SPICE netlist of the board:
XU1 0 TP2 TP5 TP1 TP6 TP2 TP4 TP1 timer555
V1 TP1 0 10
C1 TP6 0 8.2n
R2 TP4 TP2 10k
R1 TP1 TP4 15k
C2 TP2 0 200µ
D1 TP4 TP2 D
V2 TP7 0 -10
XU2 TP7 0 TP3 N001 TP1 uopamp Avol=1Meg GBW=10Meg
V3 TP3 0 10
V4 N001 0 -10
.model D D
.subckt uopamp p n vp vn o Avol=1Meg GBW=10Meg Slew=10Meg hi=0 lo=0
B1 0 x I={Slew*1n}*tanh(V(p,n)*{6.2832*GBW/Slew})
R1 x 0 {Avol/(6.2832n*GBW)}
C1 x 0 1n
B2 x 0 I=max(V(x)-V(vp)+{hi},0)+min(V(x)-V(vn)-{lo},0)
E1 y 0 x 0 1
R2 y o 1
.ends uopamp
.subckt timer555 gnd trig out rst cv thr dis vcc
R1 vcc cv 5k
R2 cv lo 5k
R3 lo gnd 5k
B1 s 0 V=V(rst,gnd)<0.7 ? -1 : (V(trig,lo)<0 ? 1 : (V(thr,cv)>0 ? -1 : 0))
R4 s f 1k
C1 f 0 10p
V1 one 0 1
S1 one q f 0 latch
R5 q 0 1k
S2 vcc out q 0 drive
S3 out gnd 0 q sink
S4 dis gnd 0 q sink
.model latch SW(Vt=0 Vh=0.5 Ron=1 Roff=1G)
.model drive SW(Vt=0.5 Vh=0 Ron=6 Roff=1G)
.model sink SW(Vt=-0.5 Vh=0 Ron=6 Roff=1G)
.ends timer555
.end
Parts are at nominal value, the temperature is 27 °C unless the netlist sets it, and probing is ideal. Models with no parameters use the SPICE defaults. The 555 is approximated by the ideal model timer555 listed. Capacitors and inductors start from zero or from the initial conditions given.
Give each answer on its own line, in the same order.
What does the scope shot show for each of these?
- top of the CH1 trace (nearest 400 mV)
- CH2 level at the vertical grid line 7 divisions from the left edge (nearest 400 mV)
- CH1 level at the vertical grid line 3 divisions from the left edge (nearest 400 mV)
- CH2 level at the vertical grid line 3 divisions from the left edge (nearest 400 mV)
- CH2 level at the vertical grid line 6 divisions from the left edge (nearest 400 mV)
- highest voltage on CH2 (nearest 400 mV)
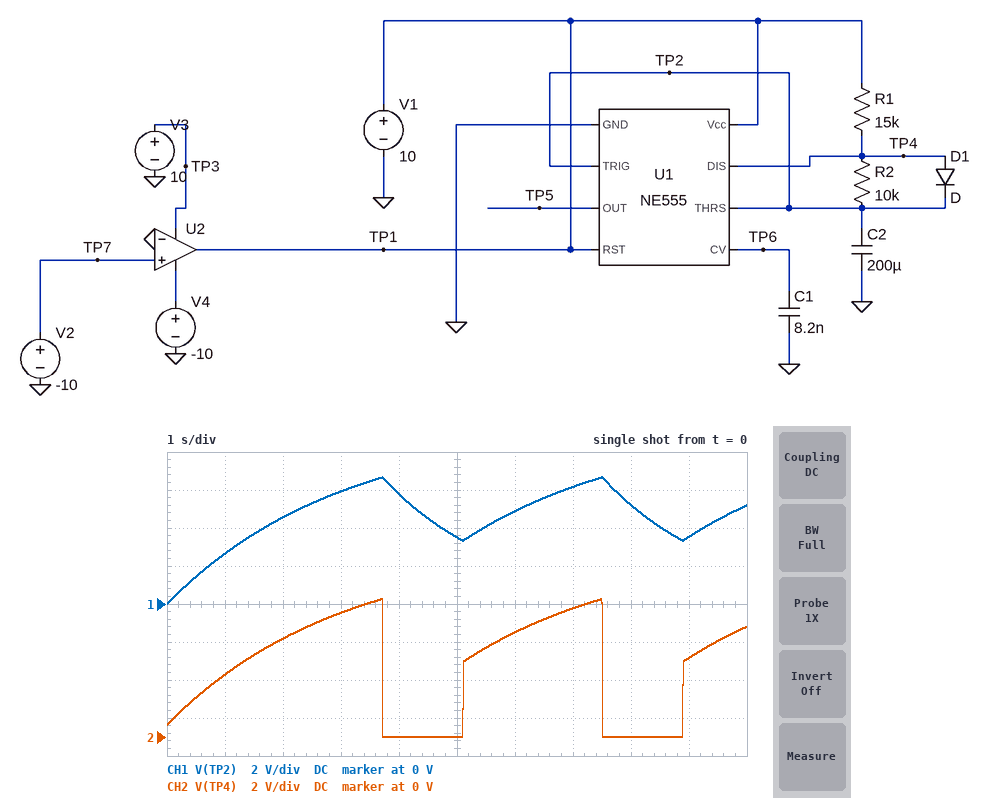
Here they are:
6.8 V
6.8 V
6.0 V
6.4 V
5.6 V
7.2 V
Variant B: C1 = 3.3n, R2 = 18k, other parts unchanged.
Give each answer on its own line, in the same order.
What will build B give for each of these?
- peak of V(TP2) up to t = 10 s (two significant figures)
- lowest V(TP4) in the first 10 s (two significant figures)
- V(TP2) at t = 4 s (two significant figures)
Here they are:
6.7 V
5.1 mV
6.2 V
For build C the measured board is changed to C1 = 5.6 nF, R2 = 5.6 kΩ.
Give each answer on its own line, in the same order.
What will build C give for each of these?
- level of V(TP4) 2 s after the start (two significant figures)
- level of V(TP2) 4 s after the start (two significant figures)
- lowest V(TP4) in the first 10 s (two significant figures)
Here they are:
5.2 V
5.2 V
7.6 mV
